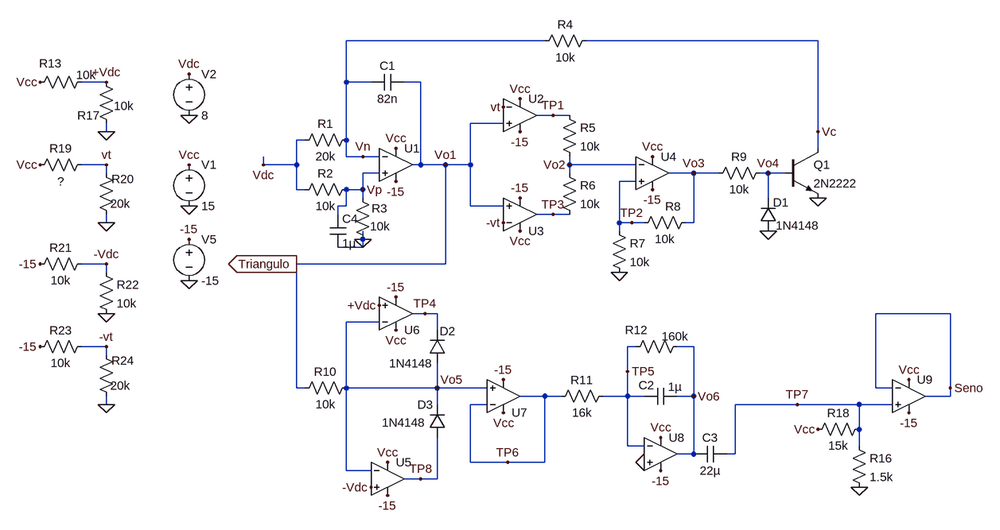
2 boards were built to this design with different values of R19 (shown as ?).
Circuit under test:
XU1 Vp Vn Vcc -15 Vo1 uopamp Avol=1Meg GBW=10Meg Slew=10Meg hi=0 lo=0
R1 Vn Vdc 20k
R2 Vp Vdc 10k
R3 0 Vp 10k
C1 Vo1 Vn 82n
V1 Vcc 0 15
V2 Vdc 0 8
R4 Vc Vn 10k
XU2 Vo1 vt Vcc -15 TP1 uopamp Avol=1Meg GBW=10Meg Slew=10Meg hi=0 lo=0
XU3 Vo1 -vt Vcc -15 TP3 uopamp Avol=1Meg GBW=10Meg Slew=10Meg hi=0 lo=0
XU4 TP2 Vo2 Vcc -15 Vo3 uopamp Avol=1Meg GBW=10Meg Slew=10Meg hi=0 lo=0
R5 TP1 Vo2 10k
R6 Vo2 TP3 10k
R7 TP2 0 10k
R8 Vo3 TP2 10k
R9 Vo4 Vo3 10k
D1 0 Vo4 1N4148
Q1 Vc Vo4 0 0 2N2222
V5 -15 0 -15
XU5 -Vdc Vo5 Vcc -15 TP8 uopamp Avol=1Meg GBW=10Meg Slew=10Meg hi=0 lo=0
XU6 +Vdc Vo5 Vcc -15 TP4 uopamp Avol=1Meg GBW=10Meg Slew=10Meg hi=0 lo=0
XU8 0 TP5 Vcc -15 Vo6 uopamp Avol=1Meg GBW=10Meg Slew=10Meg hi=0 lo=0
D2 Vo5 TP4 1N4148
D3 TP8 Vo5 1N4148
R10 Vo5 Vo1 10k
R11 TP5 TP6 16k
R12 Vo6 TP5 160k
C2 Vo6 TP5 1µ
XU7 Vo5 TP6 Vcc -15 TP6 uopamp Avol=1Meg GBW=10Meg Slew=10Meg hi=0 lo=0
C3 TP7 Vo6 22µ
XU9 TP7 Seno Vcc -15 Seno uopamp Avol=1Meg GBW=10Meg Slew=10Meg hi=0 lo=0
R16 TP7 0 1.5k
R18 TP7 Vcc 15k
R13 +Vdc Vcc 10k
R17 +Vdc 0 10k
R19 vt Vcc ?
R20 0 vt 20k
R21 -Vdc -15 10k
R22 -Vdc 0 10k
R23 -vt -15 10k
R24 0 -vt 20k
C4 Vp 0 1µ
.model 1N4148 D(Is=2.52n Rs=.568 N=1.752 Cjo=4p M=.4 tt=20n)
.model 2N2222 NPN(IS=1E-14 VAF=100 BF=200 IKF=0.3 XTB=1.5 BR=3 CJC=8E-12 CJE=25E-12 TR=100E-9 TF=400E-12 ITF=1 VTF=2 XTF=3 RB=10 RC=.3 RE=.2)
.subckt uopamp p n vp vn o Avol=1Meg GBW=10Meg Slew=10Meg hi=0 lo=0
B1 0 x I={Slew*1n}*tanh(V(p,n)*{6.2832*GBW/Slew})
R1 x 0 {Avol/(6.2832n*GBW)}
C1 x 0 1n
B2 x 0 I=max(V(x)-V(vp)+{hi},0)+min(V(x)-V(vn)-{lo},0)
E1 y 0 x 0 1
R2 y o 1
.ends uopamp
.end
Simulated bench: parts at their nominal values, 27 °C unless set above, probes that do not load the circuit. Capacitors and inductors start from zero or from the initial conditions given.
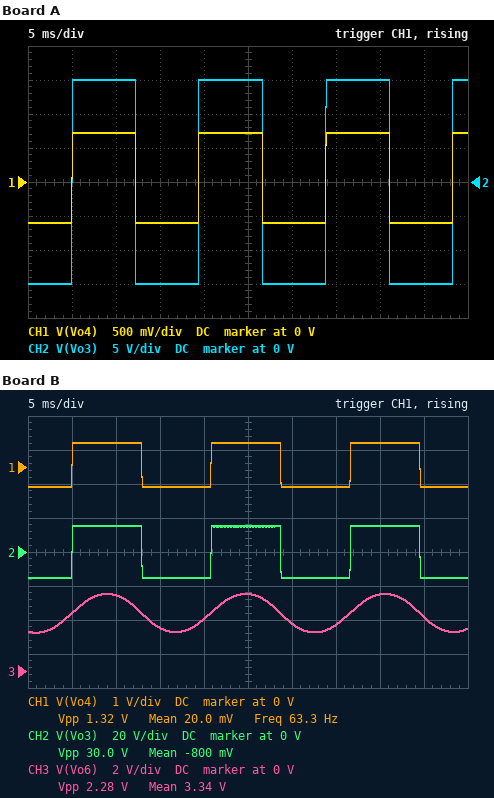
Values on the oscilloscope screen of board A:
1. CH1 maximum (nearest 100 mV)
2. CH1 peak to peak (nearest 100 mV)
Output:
700 mV
1.3 V
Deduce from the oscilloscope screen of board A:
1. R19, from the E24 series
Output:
20 kΩ
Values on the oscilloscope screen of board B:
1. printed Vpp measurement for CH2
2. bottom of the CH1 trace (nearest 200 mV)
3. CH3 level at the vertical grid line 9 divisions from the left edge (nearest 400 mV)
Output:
30.0 V
-600 mV
3.2 V
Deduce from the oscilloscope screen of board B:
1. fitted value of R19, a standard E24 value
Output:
13 kΩ
